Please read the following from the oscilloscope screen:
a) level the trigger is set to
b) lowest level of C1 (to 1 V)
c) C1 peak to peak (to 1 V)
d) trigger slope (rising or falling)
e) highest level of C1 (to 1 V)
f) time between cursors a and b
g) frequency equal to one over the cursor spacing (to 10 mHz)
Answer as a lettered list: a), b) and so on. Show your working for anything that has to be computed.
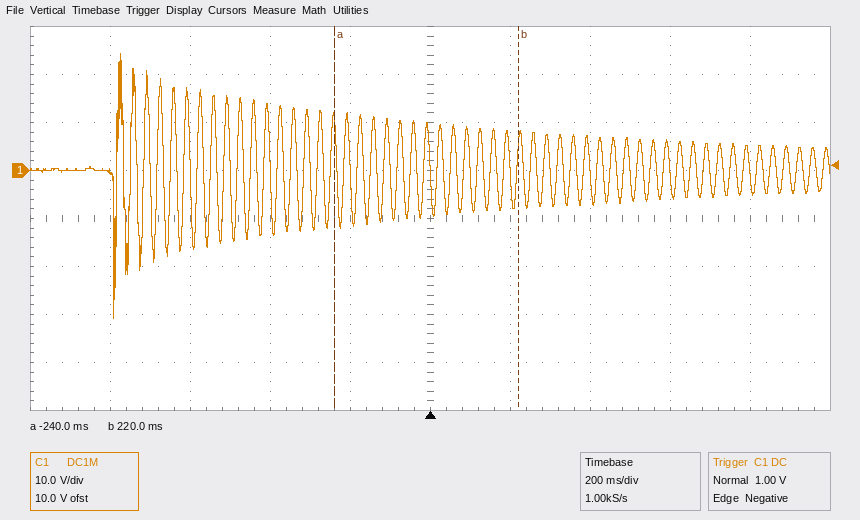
a) 1.00 V
b) -31 V
c) 24 V − (-31 V) = 55 V
d) falling
e) 24 V
f) 220 ms − (-240 ms) = 460 ms
g) 1 / 460 ms ≈ 2.17 Hz
